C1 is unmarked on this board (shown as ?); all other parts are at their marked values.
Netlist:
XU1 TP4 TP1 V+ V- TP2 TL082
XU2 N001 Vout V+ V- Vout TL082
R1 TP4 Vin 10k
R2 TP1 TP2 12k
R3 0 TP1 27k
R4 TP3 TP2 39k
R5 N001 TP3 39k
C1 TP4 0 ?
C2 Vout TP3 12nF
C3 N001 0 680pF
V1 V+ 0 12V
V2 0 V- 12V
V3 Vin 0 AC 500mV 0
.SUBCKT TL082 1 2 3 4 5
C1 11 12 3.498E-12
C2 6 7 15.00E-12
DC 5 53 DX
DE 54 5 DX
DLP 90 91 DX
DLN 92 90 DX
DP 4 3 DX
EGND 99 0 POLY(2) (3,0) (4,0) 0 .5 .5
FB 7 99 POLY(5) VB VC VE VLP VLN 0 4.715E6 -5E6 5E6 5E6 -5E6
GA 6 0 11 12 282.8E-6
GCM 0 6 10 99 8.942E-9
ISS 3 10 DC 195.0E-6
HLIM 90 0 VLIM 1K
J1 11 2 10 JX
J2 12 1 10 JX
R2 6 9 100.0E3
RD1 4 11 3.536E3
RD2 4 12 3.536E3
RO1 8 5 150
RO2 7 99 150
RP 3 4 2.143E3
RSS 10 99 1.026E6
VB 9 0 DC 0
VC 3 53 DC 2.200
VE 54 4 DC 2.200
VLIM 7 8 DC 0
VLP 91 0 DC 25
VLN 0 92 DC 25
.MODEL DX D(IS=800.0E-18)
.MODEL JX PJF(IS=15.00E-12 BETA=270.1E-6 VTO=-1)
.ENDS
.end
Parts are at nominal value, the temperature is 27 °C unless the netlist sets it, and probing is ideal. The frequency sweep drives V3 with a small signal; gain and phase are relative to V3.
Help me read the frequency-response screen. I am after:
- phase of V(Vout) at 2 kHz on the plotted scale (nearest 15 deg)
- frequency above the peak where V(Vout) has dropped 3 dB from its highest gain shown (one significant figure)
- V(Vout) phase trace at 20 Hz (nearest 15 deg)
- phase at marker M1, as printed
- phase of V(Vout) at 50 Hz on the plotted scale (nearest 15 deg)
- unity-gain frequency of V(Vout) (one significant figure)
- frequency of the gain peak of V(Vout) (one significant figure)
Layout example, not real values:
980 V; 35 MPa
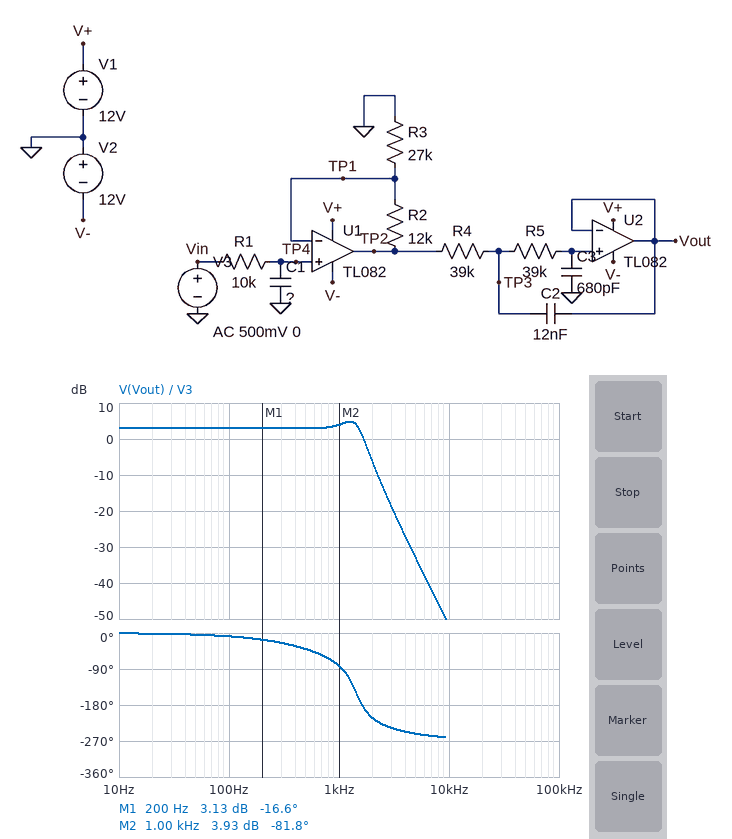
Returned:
-210 deg; 2 kHz; 0 deg; -16.6 deg; 0 deg; 2 kHz; 1 kHz
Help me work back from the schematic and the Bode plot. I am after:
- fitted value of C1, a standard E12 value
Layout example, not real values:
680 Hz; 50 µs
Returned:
18 nF
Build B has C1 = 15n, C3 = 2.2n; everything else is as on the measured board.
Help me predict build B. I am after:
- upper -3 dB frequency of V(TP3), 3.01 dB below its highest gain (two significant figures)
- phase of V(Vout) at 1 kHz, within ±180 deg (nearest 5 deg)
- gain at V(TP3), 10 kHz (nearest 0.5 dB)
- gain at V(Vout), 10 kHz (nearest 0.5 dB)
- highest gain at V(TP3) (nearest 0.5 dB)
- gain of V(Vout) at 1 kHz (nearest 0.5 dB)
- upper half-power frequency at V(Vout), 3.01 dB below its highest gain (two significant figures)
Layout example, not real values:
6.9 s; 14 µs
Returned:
900 Hz; -160 deg; -45.5 dB; -60.5 dB; 4.5 dB; -1.5 dB; 880 Hz
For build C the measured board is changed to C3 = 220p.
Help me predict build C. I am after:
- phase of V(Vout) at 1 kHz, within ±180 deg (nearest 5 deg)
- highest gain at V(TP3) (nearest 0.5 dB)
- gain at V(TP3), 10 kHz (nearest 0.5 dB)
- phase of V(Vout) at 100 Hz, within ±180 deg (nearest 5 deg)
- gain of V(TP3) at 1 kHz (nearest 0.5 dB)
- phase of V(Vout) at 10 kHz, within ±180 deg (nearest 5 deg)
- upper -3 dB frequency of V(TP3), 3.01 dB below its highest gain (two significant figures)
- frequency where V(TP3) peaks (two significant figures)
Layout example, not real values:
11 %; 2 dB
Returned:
-55 deg; 5.5 dB; -40.5 dB; -5 deg; 1.0 dB; 100 deg; 2.7 kHz; 2.4 kHz
